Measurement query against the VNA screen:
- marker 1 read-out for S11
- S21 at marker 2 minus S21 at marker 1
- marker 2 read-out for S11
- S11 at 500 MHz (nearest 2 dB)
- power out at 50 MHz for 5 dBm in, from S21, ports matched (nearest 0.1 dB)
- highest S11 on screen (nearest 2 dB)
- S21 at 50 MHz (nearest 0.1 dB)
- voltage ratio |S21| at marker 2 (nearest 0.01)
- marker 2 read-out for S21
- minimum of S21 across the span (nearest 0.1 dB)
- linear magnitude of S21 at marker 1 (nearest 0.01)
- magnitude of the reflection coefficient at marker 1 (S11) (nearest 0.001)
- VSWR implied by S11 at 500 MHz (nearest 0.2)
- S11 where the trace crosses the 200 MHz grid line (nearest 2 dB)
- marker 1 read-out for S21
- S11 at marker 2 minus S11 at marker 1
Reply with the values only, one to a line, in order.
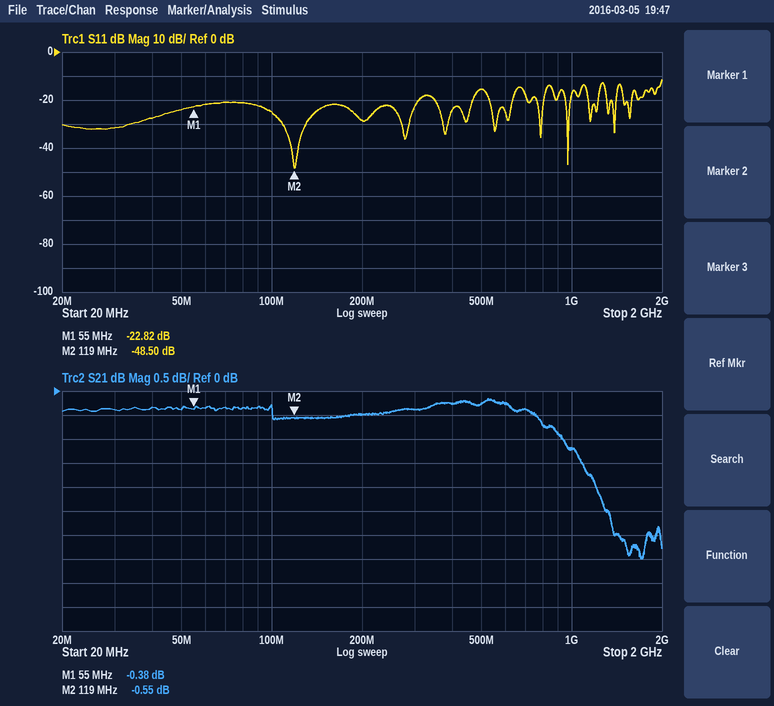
-22.82 dB
-0.17 dB
-48.50 dB
-16 dB
4.6 dBm
-12 dB
-0.4 dB
0.94
-0.55 dB
-3.5 dB
0.96
0.072
1.4
-28 dB
-0.38 dB
-25.68 dB
